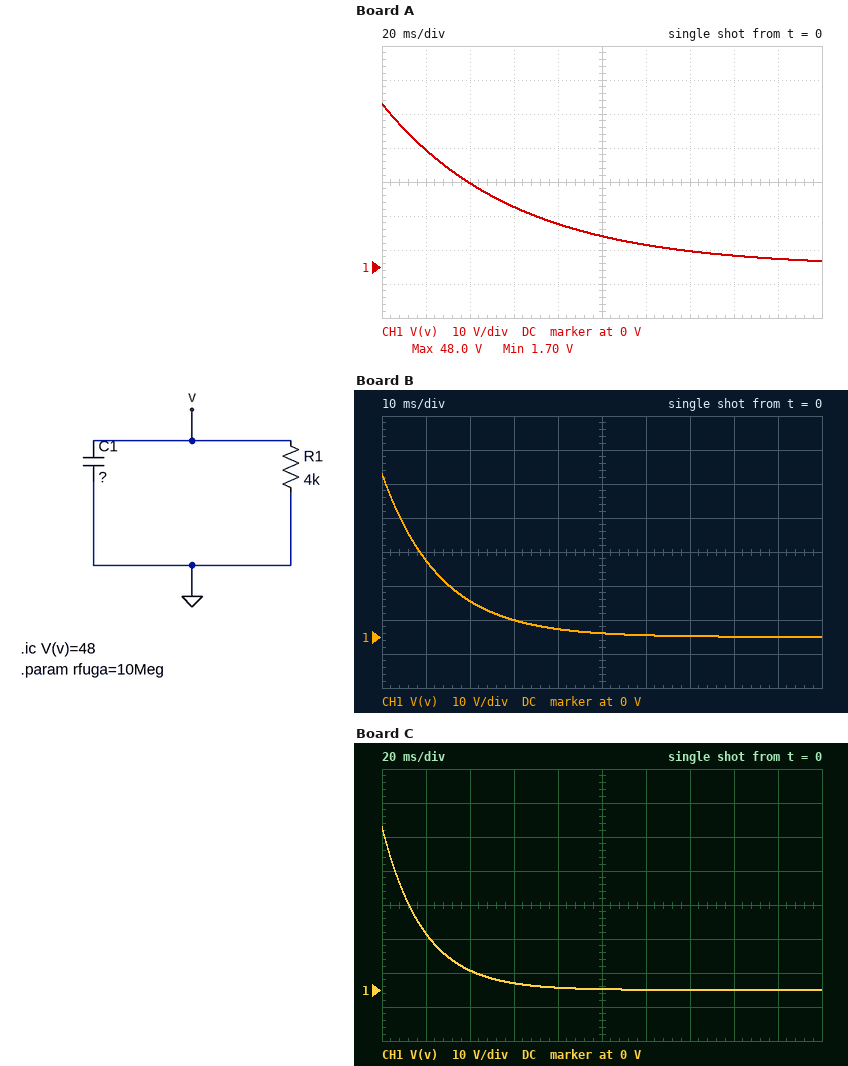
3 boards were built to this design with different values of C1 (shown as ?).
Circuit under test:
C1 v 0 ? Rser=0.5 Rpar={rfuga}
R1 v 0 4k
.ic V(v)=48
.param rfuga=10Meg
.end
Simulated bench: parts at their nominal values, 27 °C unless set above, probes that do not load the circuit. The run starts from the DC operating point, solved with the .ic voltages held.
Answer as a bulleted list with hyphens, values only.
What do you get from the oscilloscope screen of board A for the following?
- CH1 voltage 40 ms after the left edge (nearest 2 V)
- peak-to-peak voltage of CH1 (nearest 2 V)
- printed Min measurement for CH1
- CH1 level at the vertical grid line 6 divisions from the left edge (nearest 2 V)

- 24 V
- 46 V
- 1.70 V
- 6 V
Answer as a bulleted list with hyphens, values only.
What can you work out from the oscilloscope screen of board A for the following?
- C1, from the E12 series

- 15 µF
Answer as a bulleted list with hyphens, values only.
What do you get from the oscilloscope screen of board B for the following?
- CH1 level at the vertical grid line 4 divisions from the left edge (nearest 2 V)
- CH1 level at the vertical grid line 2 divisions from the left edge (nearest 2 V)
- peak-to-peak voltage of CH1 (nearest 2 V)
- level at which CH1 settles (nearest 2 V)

- 2 V
- 10 V
- 48 V
- 0 V
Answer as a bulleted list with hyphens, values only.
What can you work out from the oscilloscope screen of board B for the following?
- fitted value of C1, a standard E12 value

- 3.3 µF
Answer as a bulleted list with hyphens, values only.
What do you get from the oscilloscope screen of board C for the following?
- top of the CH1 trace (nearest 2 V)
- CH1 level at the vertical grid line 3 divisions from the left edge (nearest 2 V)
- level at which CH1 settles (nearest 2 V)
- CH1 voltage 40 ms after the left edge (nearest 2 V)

- 48 V
- 2 V
- 0 V
- 6 V
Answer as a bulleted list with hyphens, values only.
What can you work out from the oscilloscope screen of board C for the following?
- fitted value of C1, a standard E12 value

- 4.7 µF
